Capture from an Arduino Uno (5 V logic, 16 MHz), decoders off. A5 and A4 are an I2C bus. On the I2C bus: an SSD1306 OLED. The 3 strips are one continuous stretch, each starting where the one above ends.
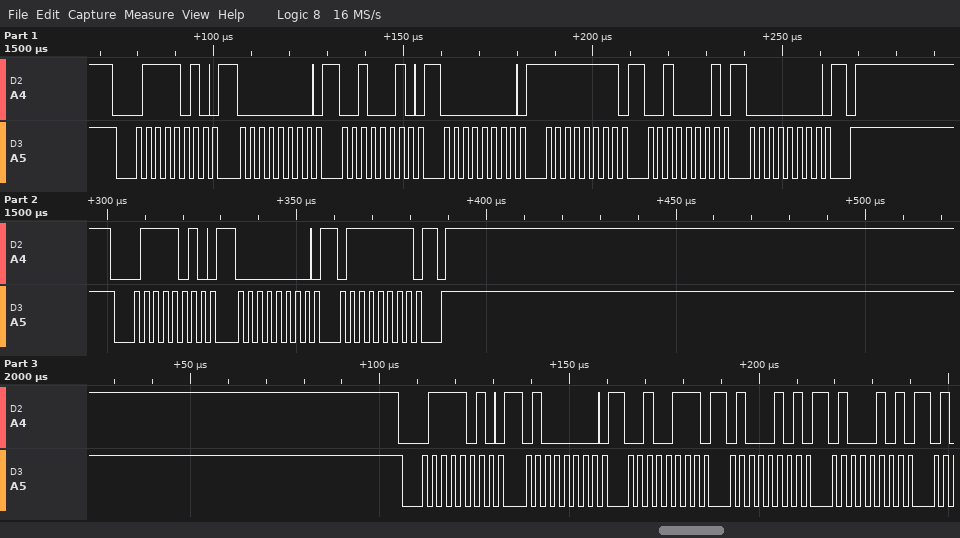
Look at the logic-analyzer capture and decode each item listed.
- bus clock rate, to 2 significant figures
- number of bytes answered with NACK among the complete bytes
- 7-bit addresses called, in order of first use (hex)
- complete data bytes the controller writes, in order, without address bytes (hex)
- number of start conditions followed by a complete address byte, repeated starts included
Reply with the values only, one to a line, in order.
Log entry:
400 kHz
0
0x3D
00 22 00 FF 21 00 00 7F 40 27 45 45
3
